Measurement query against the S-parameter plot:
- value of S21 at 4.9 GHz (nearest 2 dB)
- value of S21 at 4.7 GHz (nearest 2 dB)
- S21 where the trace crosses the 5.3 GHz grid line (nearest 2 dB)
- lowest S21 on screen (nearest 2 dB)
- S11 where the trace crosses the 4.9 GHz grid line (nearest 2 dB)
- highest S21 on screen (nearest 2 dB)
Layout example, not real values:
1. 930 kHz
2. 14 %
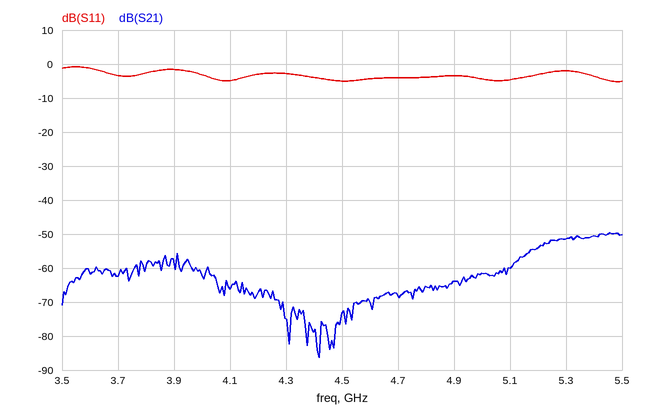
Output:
1. -64 dB
2. -68 dB
3. -52 dB
4. -86 dB
5. -4 dB
6. -50 dB
